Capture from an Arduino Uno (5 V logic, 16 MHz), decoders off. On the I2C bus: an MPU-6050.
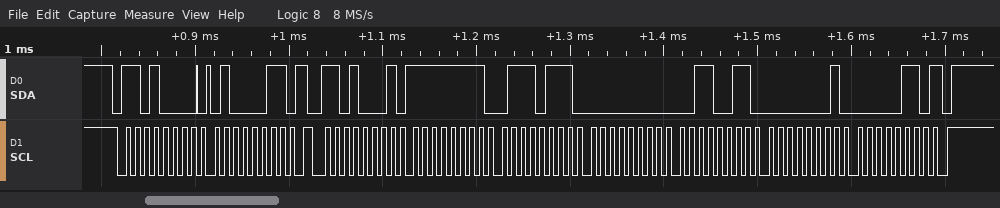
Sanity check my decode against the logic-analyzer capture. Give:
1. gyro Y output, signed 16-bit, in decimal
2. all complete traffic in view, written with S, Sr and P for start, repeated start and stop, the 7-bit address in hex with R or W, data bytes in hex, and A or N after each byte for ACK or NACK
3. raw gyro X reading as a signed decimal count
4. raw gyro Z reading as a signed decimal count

51
S 68W A 43 A Sr 68R A FF A 77 A 00 A 33 A 01 A 06 N P
-137
262
